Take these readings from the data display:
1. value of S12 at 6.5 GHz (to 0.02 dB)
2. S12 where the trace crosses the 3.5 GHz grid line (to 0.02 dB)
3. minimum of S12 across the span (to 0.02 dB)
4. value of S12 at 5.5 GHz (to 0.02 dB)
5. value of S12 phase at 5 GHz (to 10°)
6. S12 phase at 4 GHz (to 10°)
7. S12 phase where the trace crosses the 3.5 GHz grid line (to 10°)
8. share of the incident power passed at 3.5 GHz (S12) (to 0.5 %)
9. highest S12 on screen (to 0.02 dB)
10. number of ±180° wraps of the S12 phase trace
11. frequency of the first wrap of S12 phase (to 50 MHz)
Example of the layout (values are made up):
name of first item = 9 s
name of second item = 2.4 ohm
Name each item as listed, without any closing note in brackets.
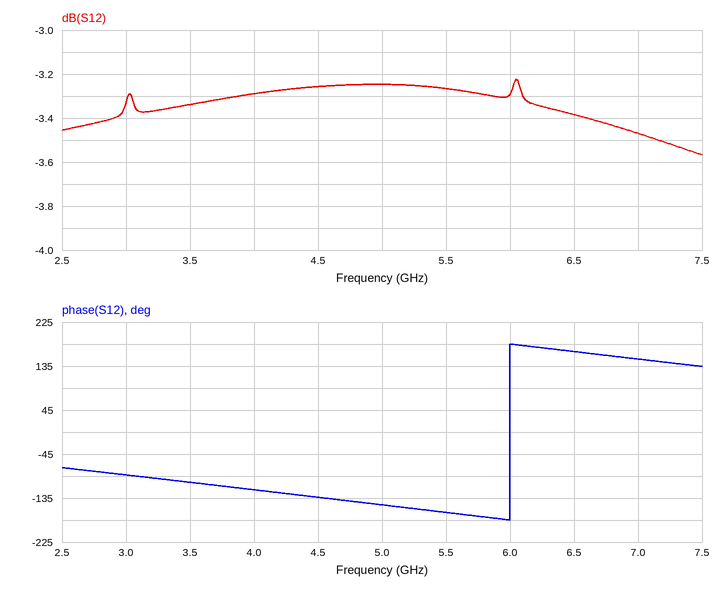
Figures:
value of S12 at 6.5 GHz = -3.38 dB
S12 where the trace crosses the 3.5 GHz grid line = -3.34 dB
minimum of S12 across the span = -3.56 dB
value of S12 at 5.5 GHz = -3.26 dB
value of S12 phase at 5 GHz = -150°
S12 phase at 4 GHz = -120°
S12 phase where the trace crosses the 3.5 GHz grid line = -100°
share of the incident power passed at 3.5 GHz (S12) = 46.5 %
highest S12 on screen = -3.22 dB
number of ±180° wraps of the S12 phase trace = 1
frequency of the first wrap of S12 phase = 6.00 GHz
